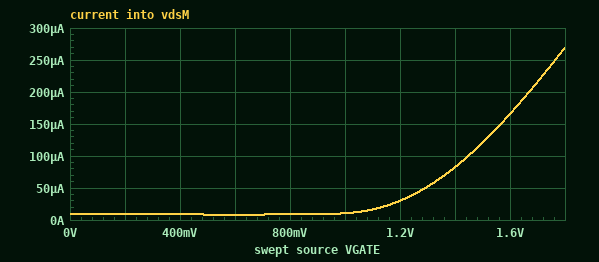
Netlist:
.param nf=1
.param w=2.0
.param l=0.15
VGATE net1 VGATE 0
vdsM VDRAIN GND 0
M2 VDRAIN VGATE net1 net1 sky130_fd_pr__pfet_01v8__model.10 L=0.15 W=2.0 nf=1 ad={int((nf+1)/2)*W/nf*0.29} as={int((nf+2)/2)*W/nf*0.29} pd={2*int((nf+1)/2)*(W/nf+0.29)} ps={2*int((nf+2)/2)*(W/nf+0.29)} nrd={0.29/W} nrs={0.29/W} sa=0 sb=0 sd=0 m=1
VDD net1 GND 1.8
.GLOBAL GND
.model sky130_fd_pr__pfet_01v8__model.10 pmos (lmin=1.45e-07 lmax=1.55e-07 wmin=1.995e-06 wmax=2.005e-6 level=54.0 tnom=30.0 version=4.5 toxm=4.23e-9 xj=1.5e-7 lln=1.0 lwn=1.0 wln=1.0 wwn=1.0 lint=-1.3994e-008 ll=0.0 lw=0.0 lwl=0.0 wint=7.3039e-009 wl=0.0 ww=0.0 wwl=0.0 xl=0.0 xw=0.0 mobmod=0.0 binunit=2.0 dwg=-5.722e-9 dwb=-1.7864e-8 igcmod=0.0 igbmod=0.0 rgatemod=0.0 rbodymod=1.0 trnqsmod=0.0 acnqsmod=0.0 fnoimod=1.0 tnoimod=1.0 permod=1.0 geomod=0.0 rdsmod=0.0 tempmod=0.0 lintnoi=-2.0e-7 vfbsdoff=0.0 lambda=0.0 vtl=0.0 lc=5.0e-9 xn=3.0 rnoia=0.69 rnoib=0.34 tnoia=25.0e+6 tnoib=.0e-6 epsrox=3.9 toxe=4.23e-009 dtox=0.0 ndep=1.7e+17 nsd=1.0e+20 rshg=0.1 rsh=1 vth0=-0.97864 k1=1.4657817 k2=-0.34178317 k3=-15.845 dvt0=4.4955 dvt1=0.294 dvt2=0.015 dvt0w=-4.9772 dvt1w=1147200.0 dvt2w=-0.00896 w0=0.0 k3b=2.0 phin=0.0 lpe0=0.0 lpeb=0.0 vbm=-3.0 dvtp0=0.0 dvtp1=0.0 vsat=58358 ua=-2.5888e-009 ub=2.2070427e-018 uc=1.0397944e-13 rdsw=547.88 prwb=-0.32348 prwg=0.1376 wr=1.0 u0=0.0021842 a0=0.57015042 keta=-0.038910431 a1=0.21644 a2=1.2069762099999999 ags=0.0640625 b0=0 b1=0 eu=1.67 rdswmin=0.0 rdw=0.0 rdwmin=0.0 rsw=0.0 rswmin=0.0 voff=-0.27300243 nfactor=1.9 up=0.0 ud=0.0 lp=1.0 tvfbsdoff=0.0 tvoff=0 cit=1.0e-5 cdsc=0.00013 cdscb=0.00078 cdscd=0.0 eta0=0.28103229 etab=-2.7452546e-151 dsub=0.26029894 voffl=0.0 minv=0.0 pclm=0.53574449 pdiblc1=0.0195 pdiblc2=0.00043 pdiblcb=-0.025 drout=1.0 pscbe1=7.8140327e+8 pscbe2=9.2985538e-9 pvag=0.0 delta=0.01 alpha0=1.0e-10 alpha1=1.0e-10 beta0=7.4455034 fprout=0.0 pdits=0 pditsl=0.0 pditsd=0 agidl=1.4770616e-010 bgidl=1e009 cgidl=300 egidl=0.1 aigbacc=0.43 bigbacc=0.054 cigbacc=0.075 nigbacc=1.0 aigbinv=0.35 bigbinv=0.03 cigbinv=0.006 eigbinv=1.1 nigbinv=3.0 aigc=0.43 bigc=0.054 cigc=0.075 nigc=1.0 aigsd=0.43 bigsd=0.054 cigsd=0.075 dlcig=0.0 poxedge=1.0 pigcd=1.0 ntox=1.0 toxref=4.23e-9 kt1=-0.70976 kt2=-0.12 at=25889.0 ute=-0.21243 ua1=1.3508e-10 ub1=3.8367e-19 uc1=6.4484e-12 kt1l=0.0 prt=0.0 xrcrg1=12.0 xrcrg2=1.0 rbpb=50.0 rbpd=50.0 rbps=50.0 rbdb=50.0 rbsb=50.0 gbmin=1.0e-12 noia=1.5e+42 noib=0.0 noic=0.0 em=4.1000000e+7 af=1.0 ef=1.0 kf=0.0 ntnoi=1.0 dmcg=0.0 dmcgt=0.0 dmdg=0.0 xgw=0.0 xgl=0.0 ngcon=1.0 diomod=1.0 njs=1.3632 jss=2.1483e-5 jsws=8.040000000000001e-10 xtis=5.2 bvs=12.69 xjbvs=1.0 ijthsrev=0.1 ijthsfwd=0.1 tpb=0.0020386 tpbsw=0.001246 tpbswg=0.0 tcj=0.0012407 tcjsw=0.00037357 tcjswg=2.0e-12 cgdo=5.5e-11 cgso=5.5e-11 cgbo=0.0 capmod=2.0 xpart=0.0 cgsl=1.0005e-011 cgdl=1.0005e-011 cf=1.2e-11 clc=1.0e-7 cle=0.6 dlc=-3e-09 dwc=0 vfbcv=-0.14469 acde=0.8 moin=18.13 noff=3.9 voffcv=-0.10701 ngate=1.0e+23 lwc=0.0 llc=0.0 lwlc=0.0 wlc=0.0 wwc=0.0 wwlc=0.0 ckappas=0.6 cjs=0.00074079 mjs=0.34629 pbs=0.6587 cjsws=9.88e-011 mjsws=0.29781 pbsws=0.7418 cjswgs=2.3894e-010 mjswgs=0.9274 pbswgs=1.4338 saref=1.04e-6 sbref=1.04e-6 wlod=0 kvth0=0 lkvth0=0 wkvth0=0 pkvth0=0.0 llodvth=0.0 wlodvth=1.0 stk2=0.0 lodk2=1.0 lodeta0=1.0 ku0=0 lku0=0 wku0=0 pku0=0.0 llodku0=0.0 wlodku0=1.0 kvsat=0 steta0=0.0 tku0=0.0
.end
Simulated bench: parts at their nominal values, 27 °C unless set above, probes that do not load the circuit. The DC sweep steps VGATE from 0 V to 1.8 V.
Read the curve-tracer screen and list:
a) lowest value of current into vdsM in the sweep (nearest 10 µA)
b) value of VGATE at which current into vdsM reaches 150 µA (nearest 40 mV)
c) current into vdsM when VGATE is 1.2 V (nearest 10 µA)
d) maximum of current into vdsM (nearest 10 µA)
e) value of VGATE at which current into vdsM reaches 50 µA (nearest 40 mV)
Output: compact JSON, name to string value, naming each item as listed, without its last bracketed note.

{"lowest value of current into vdsM in the sweep": "10 µA", "value of VGATE at which current into vdsM reaches 150 µA": "1.56 V", "current into vdsM when VGATE is 1.2 V": "30 µA", "maximum of current into vdsM": "270 µA", "value of VGATE at which current into vdsM reaches 50 µA": "1.28 V"}
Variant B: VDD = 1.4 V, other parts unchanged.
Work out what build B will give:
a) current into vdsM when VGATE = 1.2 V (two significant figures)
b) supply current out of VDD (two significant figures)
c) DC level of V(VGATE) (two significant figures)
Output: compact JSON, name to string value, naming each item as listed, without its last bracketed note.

{"current into vdsM when VGATE = 1.2 V": "30 µA", "supply current out of VDD": "8.6 µA", "DC level of V(VGATE)": "1.4 V"}
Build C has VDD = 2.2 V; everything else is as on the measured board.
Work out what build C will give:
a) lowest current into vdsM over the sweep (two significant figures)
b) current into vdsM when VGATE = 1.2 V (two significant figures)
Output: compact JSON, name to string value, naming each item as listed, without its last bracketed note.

{"lowest current into vdsM over the sweep": "8.7 µA", "current into vdsM when VGATE = 1.2 V": "30 µA"}
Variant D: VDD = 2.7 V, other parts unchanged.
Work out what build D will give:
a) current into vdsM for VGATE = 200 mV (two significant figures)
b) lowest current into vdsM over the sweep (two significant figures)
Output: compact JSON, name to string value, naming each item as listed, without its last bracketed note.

{"current into vdsM for VGATE = 200 mV": "26 µA", "lowest current into vdsM over the sweep": "10 µA"}
